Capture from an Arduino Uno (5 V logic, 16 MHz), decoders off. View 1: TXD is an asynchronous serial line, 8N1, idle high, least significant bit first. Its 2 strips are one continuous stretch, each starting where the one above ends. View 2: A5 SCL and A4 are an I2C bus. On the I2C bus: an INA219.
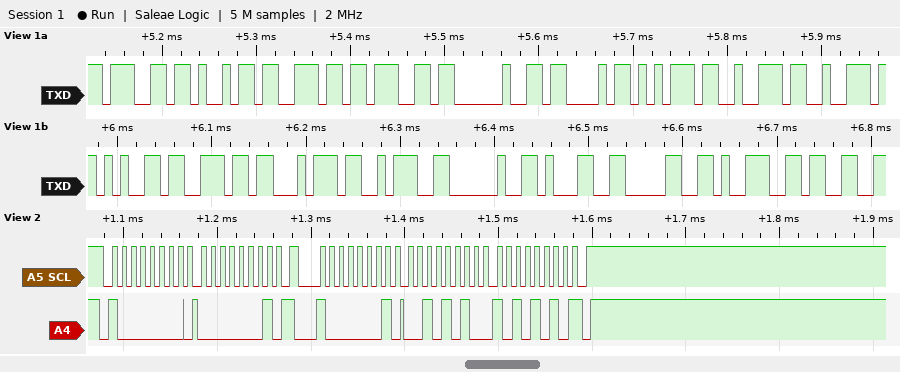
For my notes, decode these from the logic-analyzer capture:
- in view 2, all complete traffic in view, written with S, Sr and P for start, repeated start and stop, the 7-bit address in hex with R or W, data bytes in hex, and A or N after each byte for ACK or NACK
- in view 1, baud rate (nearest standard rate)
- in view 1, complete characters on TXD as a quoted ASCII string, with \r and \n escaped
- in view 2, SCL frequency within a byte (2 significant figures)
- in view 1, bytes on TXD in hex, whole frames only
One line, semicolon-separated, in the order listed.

S 40W A 01 A Sr 40R A 2A A AA N P; 115200 baud; "ging Current: 1093"; 100 kHz; 67 69 6E 67 20 43 75 72 72 65 6E 74 3A 20 31 30 39 33
